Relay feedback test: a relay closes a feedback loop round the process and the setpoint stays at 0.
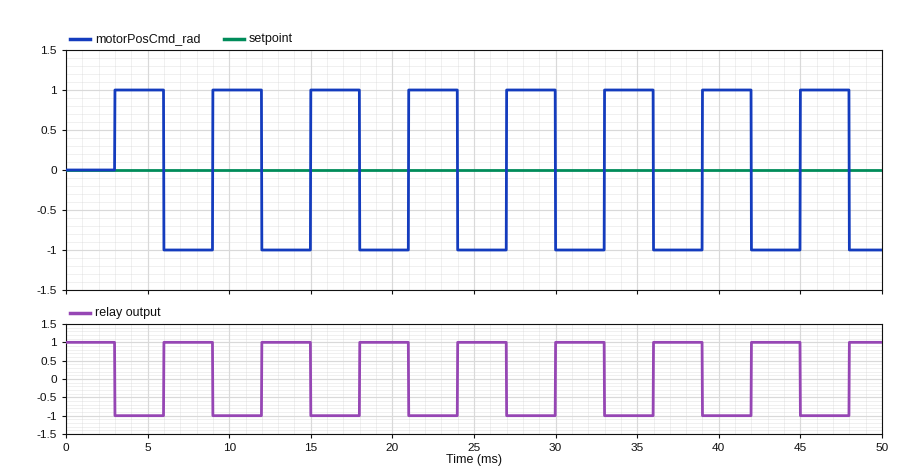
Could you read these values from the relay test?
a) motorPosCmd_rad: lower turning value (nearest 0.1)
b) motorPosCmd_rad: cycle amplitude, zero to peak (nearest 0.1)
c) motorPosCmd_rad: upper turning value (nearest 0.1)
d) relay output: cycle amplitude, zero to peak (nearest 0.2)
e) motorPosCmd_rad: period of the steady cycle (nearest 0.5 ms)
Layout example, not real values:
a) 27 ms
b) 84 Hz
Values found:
a) -1.0
b) 1.0
c) 1.0
d) 1.0
e) 6.0 ms
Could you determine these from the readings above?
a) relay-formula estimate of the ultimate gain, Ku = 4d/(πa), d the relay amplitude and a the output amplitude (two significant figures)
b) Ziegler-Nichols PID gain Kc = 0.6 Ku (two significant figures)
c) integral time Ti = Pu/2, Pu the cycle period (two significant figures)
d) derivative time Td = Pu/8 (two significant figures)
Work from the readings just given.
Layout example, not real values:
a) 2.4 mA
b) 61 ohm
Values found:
a) 1.3
b) 0.78
c) 3.0 ms
d) 0.75 ms
